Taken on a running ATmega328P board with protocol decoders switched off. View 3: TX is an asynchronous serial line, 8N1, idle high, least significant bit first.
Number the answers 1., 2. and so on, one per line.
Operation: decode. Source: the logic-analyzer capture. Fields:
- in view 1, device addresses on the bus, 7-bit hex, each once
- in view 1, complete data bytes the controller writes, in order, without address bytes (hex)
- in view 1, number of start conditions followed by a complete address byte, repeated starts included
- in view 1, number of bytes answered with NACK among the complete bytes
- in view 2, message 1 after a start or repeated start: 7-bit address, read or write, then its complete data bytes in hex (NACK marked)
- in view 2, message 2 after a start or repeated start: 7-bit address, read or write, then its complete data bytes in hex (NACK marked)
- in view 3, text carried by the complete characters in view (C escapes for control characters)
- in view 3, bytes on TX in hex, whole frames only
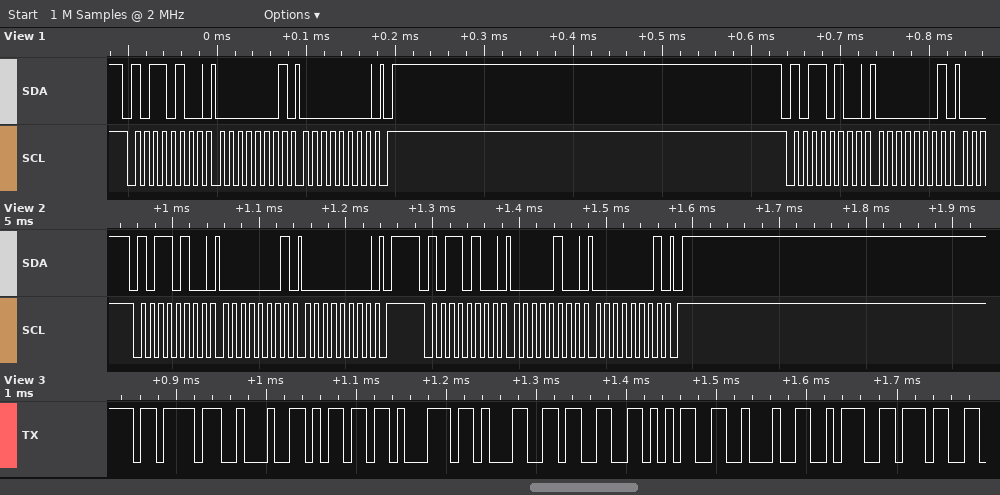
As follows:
1. 0x5A
2. 01 00 01
3. 2
4. 0
5. 0x5A write: 01 00
6. 0x5A write: 04 01
7. "{\"mq135\":7"
8. 7B 22 6D 71 31 33 35 22 3A 37
